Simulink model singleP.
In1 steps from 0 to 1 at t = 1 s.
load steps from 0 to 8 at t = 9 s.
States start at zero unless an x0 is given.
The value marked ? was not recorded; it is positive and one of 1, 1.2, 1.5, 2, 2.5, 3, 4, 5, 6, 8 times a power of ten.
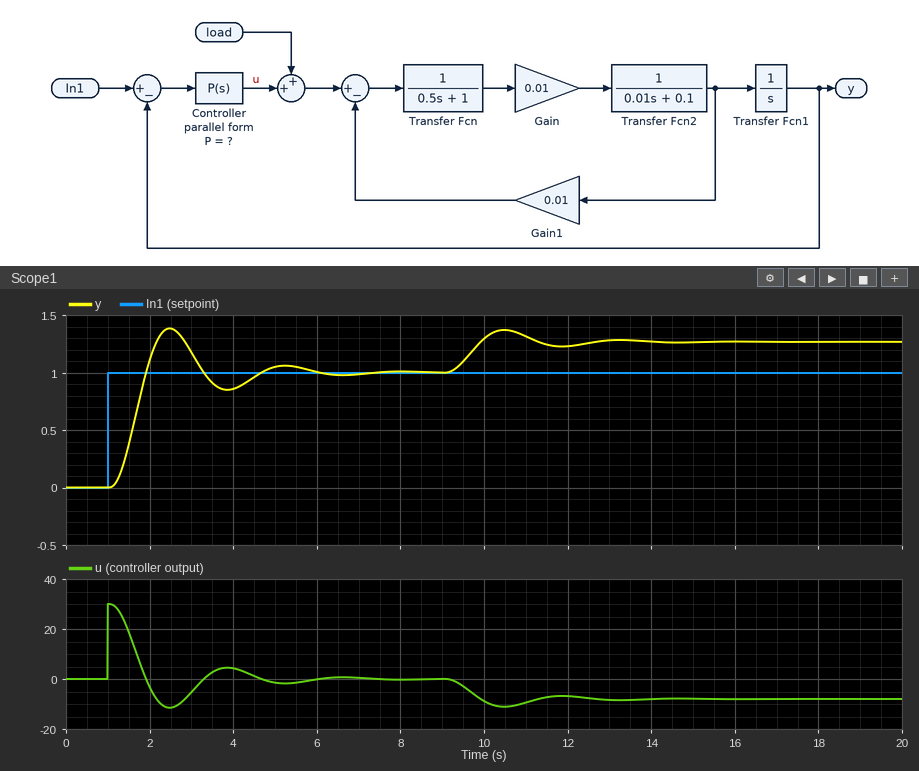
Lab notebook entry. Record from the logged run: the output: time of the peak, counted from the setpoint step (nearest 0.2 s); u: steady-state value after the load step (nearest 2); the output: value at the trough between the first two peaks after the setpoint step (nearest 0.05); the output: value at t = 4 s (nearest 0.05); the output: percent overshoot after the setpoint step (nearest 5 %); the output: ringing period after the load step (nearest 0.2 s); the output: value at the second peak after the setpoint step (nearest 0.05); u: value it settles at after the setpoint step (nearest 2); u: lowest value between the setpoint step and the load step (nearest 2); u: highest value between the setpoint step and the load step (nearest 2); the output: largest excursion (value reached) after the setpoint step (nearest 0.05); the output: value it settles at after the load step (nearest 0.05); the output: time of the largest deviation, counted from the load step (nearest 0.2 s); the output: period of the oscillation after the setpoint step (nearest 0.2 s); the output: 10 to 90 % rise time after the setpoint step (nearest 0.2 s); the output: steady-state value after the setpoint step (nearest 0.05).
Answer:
1.4 s
-8
0.85
0.85
40 %
2.8 s
1.05
0
-12
30
1.40
1.25
1.4 s
2.8 s
0.6 s
1.00
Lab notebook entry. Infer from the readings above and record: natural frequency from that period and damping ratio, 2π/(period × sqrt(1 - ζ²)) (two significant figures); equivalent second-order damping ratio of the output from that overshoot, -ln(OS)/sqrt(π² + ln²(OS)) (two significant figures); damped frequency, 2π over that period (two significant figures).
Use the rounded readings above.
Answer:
2.3 rad/s
0.28
2.2 rad/s
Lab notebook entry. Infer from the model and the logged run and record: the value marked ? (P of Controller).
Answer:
30
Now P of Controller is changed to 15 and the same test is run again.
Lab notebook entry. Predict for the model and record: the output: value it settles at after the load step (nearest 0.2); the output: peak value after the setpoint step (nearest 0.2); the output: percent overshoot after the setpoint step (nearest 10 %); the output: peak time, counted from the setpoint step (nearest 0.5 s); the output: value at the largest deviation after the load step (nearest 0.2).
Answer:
1.6
1.2
20 %
2.0 s
1.6
